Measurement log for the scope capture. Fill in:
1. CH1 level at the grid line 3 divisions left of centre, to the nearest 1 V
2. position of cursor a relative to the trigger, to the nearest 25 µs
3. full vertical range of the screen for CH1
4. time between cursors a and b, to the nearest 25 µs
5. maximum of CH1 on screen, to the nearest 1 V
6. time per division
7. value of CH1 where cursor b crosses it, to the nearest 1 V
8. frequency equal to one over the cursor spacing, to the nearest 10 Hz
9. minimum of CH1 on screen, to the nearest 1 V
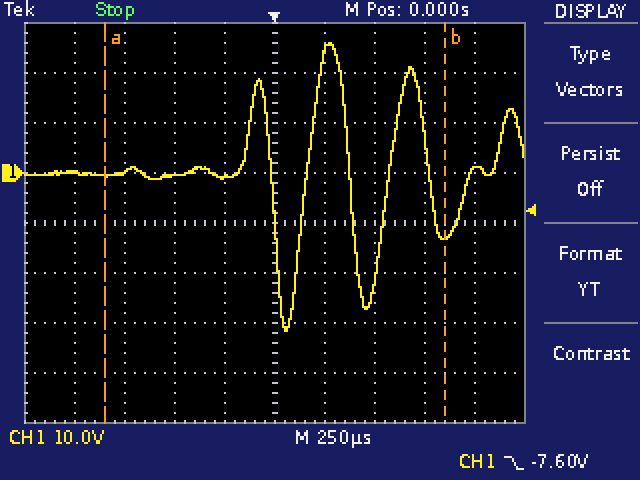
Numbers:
0 V
-850 µs
80 V
1.700 ms
26 V
250 µs
-12 V
590 Hz
-32 V
